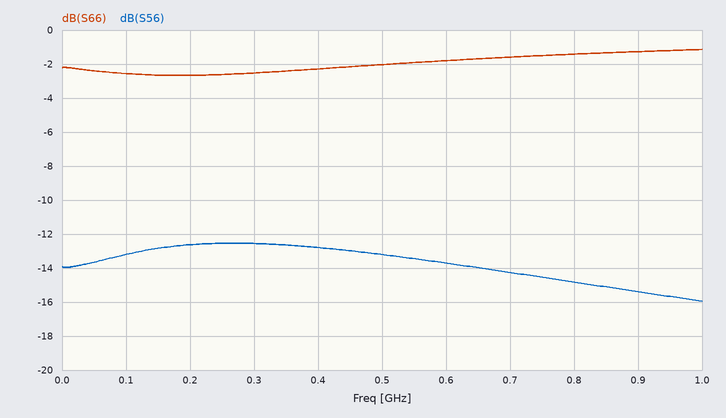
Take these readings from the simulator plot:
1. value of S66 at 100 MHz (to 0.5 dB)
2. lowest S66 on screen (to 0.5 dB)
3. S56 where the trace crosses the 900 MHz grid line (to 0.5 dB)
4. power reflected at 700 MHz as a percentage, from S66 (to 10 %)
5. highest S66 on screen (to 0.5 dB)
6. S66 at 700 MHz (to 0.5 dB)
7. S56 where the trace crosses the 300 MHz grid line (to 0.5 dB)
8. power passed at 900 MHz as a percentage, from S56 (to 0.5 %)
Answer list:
-2.5 dB
-2.5 dB
-15.5 dB
70 %
-1.0 dB
-1.5 dB
-12.5 dB
3.0 %
